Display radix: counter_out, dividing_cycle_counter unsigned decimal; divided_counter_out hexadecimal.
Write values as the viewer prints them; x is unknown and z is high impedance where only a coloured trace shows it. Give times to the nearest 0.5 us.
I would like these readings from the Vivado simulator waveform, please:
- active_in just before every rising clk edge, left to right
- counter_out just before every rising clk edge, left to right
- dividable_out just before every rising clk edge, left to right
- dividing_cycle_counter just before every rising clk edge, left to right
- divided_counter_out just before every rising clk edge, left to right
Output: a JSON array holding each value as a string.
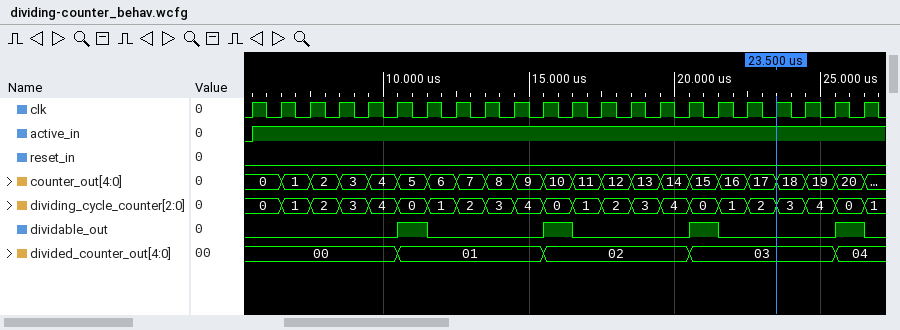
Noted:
["0 1 1 1 1 1 1 1 1 1 1 1 1 1 1 1 1 1 1 1 1 1", "0, 0, 1, 2, 3, 4, 5, 6, 7, 8, 9, 10, 11, 12, 13, 14, 15, 16, 17, 18, 19, 20", "0 0 0 0 0 0 1 0 0 0 0 1 0 0 0 0 1 0 0 0 0 1", "0, 0, 1, 2, 3, 4, 0, 1, 2, 3, 4, 0, 1, 2, 3, 4, 0, 1, 2, 3, 4, 0", "00, 00, 00, 00, 00, 00, 01, 01, 01, 01, 01, 02, 02, 02, 02, 02, 03, 03, 03, 03, 03, 04"]
